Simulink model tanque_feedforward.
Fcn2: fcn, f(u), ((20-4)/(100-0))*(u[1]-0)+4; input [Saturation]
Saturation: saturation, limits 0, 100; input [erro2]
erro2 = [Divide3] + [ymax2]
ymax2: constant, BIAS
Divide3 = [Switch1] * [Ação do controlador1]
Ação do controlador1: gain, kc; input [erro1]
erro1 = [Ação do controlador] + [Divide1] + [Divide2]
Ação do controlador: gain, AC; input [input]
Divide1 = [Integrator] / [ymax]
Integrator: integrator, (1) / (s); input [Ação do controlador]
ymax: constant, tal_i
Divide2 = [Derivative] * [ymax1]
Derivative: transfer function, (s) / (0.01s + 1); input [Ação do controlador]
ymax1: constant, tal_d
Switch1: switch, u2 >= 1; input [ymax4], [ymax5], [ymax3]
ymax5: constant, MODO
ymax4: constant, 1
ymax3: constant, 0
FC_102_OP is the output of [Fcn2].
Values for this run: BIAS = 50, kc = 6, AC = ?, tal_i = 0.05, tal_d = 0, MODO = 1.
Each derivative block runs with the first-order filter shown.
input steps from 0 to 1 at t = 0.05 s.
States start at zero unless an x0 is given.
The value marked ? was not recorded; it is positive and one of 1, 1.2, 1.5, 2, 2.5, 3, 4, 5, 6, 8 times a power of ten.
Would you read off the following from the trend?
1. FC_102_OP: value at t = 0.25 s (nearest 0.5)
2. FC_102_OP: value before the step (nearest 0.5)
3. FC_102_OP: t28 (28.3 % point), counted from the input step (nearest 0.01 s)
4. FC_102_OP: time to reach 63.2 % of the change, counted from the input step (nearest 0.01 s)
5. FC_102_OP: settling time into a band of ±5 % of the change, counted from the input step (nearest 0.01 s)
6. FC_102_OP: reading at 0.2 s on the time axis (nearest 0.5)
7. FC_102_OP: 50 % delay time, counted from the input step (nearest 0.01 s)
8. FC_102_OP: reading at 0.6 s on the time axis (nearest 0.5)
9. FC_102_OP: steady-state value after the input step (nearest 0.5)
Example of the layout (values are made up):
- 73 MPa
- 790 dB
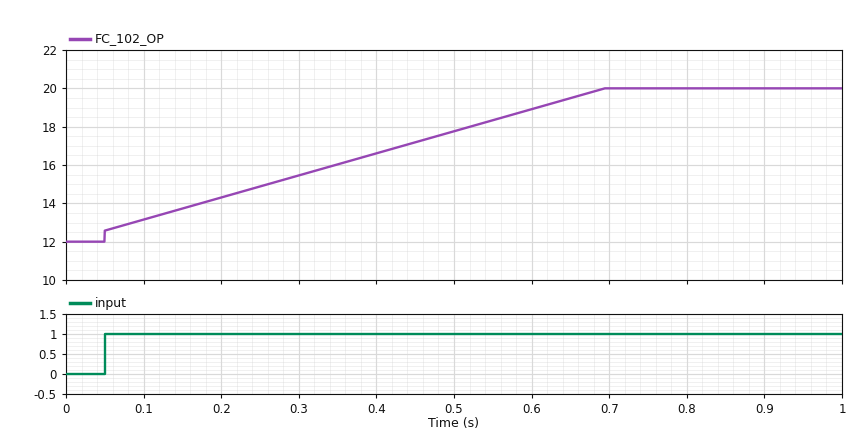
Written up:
- 15.0
- 12.0
- 0.15 s
- 0.39 s
- 0.61 s
- 14.5
- 0.30 s
- 19.0
- 20.0
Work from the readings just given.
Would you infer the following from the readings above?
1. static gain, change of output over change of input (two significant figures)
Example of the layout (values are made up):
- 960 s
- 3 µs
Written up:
- 8.0
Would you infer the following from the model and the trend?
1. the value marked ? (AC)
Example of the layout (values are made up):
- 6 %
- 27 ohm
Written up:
- 0.6
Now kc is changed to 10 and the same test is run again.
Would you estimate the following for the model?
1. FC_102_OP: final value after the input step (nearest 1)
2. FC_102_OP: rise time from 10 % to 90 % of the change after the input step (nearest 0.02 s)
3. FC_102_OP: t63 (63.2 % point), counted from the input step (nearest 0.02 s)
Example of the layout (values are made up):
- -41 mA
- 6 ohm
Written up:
- 20
- 0.32 s
- 0.22 s
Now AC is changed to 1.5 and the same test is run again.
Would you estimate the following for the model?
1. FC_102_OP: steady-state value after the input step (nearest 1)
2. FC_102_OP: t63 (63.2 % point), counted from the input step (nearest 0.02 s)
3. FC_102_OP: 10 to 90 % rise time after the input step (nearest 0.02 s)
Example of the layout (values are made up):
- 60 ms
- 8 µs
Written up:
- 20
- 0.12 s
- 0.20 s
